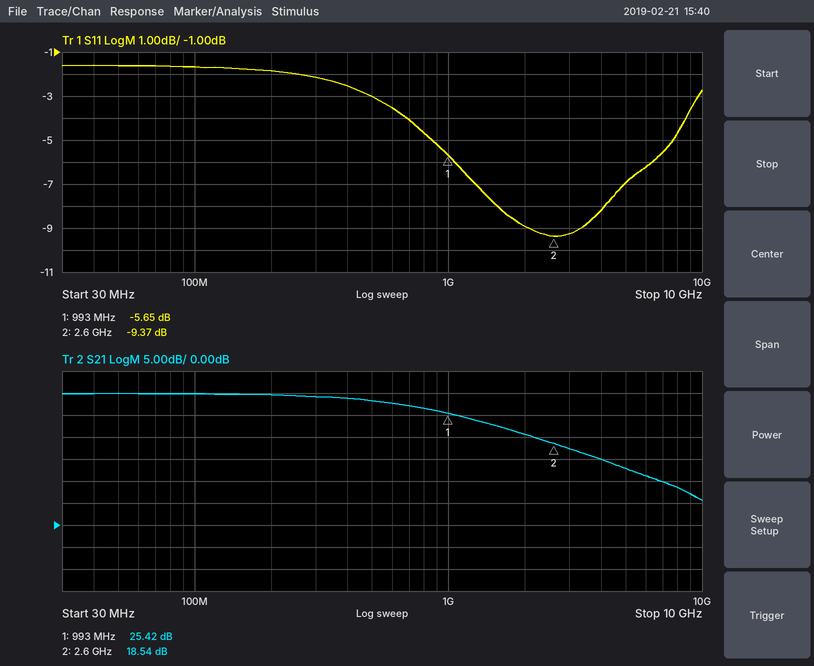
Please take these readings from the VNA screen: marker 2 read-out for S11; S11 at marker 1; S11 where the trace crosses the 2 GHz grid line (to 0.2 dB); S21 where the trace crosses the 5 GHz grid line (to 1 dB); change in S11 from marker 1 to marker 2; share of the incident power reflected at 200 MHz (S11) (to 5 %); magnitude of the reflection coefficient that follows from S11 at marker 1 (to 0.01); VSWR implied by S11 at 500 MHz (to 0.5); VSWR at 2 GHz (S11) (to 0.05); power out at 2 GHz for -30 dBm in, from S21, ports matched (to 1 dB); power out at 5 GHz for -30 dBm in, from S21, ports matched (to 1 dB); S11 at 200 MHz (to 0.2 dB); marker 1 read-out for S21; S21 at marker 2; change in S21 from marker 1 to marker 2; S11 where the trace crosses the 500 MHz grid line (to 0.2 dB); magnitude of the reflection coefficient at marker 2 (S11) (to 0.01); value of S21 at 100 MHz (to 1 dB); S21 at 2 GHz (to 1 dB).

-9.37 dB
-5.65 dB
-9.0 dB
13 dB
-3.72 dB
65 %
0.52
6.0
2.10
-9 dBm
-17 dBm
-1.8 dB
25.42 dB
18.54 dB
-6.88 dB
-3.0 dB
0.34
30 dB
21 dB
